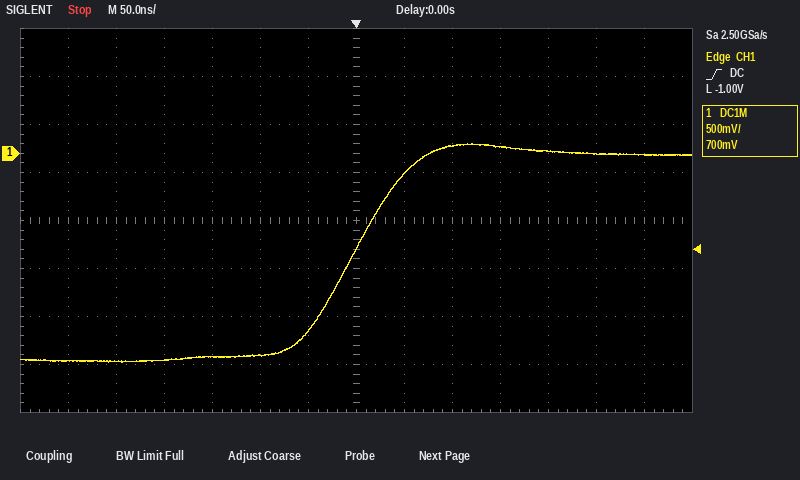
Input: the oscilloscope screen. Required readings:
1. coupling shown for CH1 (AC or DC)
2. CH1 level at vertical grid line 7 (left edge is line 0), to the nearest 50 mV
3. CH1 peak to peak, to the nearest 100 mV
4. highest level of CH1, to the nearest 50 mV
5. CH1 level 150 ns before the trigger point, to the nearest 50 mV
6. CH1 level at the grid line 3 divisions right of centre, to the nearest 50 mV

DC
-1.00 V
2.30 V
100 mV
-2.10 V
50 mV
